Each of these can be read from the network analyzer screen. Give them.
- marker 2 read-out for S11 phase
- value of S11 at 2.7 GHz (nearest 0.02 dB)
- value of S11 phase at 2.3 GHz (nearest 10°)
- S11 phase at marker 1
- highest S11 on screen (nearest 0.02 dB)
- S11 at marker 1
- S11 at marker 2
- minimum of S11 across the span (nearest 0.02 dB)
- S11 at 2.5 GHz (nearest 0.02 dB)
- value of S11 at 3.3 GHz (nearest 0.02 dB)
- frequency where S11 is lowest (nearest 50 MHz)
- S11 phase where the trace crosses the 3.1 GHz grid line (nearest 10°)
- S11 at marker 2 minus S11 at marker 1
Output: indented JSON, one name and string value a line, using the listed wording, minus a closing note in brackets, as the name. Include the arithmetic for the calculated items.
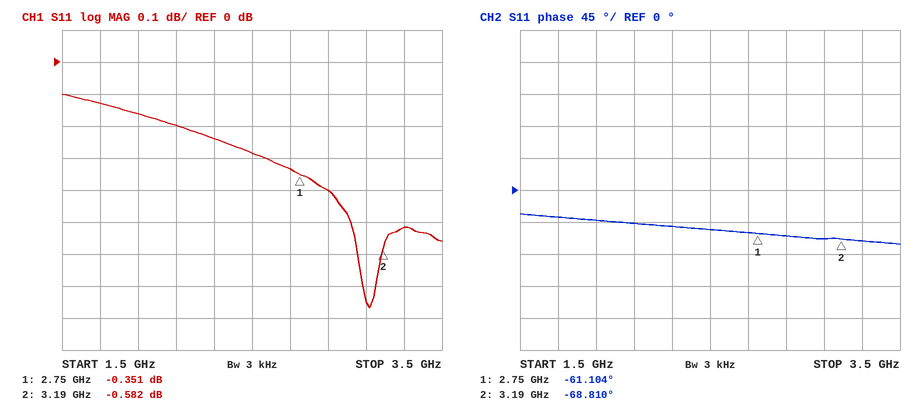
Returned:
{
  "marker 2 read-out for S11 phase": "-68.810°",
  "value of S11 at 2.7 GHz": "-0.34 dB",
  "value of S11 phase at 2.3 GHz": "-50°",
  "S11 phase at marker 1": "-61.104°",
  "highest S11 on screen": "-0.10 dB",
  "S11 at marker 1": "-0.351 dB",
  "S11 at marker 2": "-0.582 dB",
  "minimum of S11 across the span": "-0.76 dB",
  "S11 at 2.5 GHz": "-0.28 dB",
  "value of S11 at 3.3 GHz": "-0.52 dB",
  "frequency where S11 is lowest": "3.10 GHz",
  "S11 phase where the trace crosses the 3.1 GHz grid line": "-70°",
  "S11 at marker 2 minus S11 at marker 1": "-0.582 − (-0.351) = -0.231 dB"
}
